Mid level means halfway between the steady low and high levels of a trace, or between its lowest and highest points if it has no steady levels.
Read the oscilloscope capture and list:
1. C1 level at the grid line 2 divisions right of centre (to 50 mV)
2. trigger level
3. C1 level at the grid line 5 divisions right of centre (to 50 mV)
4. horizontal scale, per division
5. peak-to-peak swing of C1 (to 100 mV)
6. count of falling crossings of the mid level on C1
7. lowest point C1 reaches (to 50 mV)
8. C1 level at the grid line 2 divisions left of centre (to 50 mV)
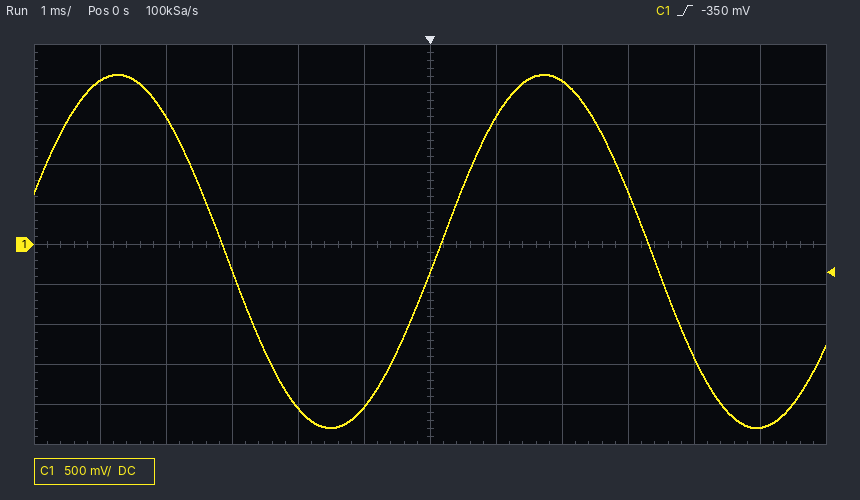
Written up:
2.05 V
-350 mV
-2.30 V
1 ms
4.40 V
2
-2.30 V
-2.05 V
